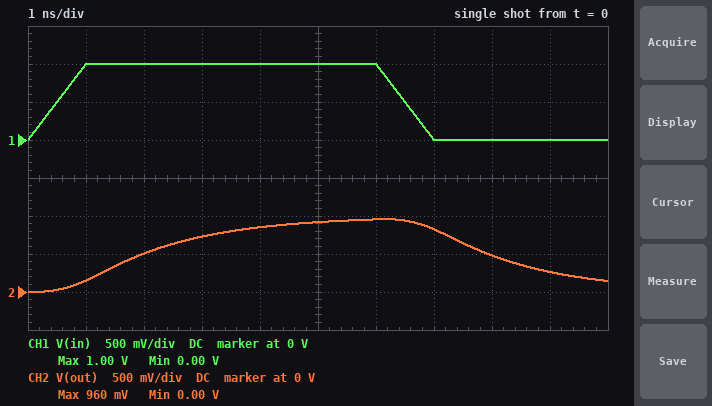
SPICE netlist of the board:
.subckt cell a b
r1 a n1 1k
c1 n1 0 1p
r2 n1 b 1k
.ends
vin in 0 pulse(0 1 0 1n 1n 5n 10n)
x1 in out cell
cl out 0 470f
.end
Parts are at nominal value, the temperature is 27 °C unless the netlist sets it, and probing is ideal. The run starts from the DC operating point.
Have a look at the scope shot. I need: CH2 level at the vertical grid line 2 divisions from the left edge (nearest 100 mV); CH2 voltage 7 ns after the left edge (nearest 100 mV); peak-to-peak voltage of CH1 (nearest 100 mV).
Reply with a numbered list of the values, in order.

1. 500 mV
2. 800 mV
3. 1.0 V
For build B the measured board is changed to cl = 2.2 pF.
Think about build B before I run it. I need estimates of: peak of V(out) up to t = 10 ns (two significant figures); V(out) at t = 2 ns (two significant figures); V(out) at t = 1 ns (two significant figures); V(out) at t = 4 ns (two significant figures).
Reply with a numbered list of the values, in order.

1. 670 mV
2. 190 mV
3. 44 mV
4. 460 mV
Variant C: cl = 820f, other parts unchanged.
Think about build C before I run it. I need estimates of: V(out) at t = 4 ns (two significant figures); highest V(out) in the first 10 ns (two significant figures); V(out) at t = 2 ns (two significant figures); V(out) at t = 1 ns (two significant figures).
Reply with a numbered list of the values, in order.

1. 740 mV
2. 900 mV
3. 380 mV
4. 100 mV
